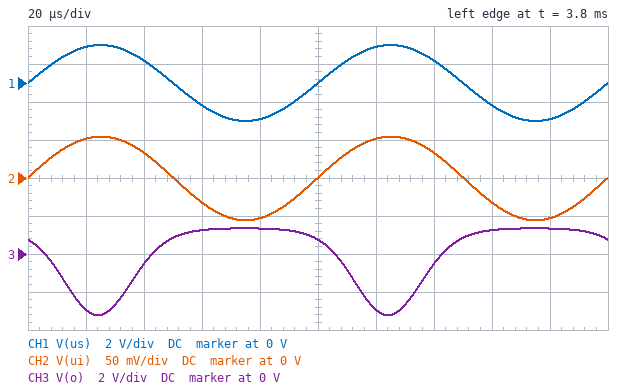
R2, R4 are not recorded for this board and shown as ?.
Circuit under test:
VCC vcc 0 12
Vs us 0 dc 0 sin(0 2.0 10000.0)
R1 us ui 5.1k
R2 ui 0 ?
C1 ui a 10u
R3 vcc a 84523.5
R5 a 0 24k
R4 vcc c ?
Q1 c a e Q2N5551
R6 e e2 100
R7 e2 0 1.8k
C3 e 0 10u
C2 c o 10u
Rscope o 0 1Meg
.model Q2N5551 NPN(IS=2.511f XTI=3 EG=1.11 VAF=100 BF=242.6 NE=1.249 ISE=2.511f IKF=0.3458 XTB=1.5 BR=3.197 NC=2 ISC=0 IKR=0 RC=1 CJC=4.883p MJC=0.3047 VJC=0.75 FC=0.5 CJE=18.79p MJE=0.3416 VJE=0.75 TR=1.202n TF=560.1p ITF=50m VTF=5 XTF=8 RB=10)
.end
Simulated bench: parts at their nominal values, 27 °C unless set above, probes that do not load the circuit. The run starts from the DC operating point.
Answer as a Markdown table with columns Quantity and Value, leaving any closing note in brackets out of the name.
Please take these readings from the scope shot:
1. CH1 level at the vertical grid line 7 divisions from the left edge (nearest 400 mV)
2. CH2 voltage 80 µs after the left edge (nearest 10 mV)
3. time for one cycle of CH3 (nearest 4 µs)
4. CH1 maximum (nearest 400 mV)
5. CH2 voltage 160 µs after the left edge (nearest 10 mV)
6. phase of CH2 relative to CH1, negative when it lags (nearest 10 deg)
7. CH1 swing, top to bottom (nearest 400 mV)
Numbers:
| Quantity | Value |
|---|---|
| CH1 level at the vertical grid line 7 divisions from the left edge | 1.2 V |
| CH2 voltage 80 µs after the left edge | -50 mV |
| time for one cycle of CH3 | 100 µs |
| CH1 maximum | 2.0 V |
| CH2 voltage 160 µs after the left edge | -30 mV |
| phase of CH2 relative to CH1, negative when it lags | 0 deg |
| CH1 swing, top to bottom | 4.0 V |
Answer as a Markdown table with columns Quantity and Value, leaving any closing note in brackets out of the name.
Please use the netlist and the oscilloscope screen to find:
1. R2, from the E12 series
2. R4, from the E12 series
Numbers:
| Quantity | Value |
|---|---|
| R2, from the E12 series | 150 Ω |
| R4, from the E12 series | 1.5 kΩ |
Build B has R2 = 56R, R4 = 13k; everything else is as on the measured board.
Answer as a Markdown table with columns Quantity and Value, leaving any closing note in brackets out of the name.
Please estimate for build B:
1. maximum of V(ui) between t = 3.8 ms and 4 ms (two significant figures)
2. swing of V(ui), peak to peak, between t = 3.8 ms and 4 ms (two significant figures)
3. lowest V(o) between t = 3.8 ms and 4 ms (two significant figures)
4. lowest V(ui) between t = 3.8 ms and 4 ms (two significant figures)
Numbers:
| Quantity | Value |
|---|---|
| maximum of V(ui) between t = 3.8 ms and 4 ms | 13 mV |
| swing of V(ui), peak to peak, between t = 3.8 ms and 4 ms | 34 mV |
| lowest V(o) between t = 3.8 ms and 4 ms | -69 mV |
| lowest V(ui) between t = 3.8 ms and 4 ms | -21 mV |
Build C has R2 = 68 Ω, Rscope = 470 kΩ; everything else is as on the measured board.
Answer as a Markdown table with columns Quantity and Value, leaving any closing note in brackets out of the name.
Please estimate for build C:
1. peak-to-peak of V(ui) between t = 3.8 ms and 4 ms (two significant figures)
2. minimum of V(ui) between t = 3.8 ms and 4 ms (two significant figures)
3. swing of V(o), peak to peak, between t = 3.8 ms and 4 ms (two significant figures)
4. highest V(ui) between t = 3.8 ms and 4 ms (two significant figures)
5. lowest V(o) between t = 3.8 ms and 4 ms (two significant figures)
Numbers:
| Quantity | Value |
|---|---|
| peak-to-peak of V(ui) between t = 3.8 ms and 4 ms | 52 mV |
| minimum of V(ui) between t = 3.8 ms and 4 ms | -26 mV |
| swing of V(o), peak to peak, between t = 3.8 ms and 4 ms | 2.6 V |
| highest V(ui) between t = 3.8 ms and 4 ms | 26 mV |
| lowest V(o) between t = 3.8 ms and 4 ms | -1.6 V |
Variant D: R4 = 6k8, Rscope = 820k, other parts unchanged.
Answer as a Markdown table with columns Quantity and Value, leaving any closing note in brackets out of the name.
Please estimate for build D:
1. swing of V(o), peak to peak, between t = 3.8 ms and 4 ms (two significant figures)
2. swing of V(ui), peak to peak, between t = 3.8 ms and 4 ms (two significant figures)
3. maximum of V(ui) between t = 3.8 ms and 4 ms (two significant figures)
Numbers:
| Quantity | Value |
|---|---|
| swing of V(o), peak to peak, between t = 3.8 ms and 4 ms | 9.4 V |
| swing of V(ui), peak to peak, between t = 3.8 ms and 4 ms | 85 mV |
| maximum of V(ui) between t = 3.8 ms and 4 ms | 30 mV |
